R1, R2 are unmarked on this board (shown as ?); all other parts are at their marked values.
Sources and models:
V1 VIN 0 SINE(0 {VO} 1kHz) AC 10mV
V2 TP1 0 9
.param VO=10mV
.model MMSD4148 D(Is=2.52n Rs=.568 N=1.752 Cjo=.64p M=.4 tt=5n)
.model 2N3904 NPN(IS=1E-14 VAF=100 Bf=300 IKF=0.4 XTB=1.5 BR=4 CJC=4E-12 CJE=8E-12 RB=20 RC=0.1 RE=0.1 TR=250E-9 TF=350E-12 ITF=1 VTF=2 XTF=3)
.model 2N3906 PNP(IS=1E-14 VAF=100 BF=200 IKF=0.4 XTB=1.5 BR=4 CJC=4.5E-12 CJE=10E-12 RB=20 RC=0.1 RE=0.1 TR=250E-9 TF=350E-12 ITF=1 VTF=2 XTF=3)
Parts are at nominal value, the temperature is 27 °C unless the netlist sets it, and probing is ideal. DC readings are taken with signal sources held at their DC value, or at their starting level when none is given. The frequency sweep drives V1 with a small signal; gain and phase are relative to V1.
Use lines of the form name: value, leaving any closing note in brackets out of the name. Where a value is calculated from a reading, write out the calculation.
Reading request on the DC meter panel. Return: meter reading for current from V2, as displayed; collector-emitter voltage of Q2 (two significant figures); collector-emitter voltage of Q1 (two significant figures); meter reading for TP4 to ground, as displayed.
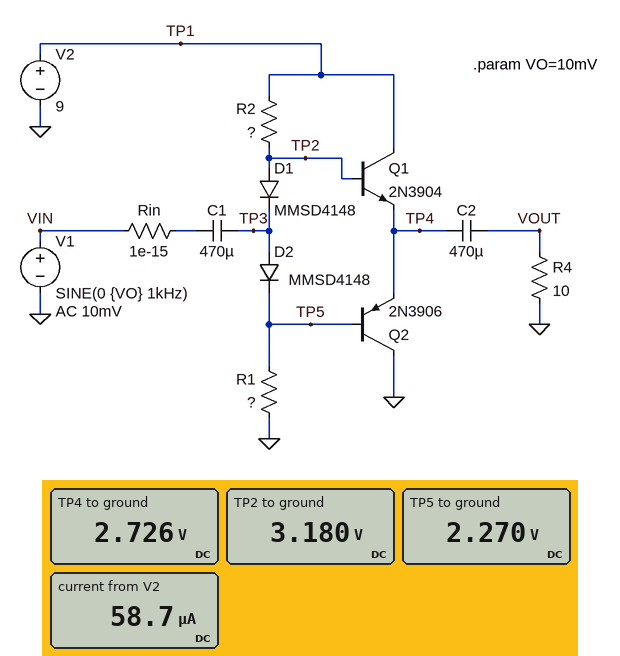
meter reading for current from V2, as displayed: 58.7 µA
collector-emitter voltage of Q2: 0 V - 2.726 V = -2.7 V
collector-emitter voltage of Q1: 9 V - 2.726 V = 6.3 V
meter reading for TP4 to ground, as displayed: 2.726 V
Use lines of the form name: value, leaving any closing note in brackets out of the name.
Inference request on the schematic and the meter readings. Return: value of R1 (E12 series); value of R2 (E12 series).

value of R1: 39 kΩ
value of R2: 100 kΩ
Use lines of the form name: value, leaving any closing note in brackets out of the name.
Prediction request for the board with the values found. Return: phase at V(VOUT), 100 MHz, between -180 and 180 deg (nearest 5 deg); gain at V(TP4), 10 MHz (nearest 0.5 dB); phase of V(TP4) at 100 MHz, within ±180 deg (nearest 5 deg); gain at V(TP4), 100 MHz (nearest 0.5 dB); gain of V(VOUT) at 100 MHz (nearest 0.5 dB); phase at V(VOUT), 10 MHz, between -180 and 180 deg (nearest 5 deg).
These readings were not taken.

phase at V(VOUT), 100 MHz, between -180 and 180 deg: 70 deg
gain at V(TP4), 10 MHz: -39.5 dB
phase of V(TP4) at 100 MHz, within ±180 deg: 70 deg
gain at V(TP4), 100 MHz: -26.0 dB
gain of V(VOUT) at 100 MHz: -26.0 dB
phase at V(VOUT), 10 MHz, between -180 and 180 deg: 60 deg
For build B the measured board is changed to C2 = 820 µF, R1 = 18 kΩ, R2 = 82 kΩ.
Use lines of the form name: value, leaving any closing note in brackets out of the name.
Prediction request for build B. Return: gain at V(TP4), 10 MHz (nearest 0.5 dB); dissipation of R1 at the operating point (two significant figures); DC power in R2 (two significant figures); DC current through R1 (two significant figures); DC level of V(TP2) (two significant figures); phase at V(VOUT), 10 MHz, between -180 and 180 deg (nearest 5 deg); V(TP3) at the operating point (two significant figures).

gain at V(TP4), 10 MHz: -38.5 dB
dissipation of R1 at the operating point: 120 µW
DC power in R2: 530 µW
DC current through R1: 81 µA
DC level of V(TP2): 2.4 V
phase at V(VOUT), 10 MHz, between -180 and 180 deg: 65 deg
V(TP3) at the operating point: 1.9 V
